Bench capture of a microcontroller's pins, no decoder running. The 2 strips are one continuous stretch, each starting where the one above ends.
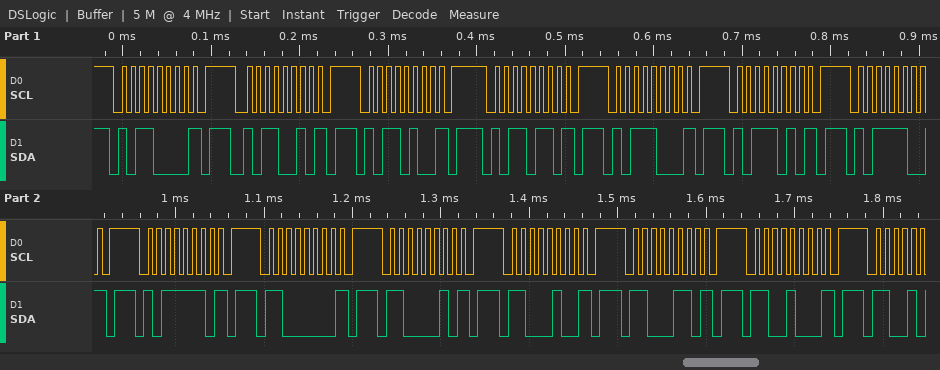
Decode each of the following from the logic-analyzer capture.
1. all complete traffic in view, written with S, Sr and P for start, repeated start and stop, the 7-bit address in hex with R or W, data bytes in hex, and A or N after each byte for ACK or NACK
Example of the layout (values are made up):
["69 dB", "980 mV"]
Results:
["S 58W N P S 59W N P S 5AW N P S 5BW N P S 5CW N P S 5DW N P S 5EW N P S 5FW N P S 60W N P S 61W N P S 62W N P S 63W N P S 64W N P"]
